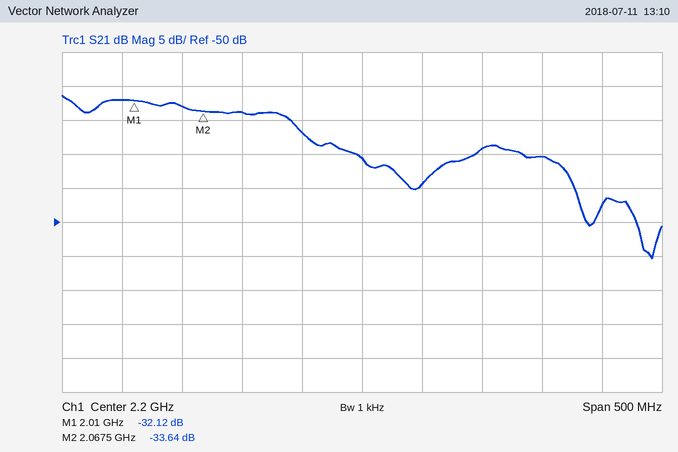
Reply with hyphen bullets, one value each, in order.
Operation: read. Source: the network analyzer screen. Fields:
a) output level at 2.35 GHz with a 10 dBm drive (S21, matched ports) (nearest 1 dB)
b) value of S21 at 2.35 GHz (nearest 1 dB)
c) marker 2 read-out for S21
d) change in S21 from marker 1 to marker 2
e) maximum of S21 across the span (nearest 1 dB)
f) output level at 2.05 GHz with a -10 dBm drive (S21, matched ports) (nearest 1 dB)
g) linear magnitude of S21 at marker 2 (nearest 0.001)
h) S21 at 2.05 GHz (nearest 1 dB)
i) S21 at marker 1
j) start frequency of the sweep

- -30 dBm
- -40 dB
- -33.64 dB
- -1.52 dB
- -31 dB
- -43 dBm
- 0.021
- -33 dB
- -32.12 dB
- 1.95 GHz
